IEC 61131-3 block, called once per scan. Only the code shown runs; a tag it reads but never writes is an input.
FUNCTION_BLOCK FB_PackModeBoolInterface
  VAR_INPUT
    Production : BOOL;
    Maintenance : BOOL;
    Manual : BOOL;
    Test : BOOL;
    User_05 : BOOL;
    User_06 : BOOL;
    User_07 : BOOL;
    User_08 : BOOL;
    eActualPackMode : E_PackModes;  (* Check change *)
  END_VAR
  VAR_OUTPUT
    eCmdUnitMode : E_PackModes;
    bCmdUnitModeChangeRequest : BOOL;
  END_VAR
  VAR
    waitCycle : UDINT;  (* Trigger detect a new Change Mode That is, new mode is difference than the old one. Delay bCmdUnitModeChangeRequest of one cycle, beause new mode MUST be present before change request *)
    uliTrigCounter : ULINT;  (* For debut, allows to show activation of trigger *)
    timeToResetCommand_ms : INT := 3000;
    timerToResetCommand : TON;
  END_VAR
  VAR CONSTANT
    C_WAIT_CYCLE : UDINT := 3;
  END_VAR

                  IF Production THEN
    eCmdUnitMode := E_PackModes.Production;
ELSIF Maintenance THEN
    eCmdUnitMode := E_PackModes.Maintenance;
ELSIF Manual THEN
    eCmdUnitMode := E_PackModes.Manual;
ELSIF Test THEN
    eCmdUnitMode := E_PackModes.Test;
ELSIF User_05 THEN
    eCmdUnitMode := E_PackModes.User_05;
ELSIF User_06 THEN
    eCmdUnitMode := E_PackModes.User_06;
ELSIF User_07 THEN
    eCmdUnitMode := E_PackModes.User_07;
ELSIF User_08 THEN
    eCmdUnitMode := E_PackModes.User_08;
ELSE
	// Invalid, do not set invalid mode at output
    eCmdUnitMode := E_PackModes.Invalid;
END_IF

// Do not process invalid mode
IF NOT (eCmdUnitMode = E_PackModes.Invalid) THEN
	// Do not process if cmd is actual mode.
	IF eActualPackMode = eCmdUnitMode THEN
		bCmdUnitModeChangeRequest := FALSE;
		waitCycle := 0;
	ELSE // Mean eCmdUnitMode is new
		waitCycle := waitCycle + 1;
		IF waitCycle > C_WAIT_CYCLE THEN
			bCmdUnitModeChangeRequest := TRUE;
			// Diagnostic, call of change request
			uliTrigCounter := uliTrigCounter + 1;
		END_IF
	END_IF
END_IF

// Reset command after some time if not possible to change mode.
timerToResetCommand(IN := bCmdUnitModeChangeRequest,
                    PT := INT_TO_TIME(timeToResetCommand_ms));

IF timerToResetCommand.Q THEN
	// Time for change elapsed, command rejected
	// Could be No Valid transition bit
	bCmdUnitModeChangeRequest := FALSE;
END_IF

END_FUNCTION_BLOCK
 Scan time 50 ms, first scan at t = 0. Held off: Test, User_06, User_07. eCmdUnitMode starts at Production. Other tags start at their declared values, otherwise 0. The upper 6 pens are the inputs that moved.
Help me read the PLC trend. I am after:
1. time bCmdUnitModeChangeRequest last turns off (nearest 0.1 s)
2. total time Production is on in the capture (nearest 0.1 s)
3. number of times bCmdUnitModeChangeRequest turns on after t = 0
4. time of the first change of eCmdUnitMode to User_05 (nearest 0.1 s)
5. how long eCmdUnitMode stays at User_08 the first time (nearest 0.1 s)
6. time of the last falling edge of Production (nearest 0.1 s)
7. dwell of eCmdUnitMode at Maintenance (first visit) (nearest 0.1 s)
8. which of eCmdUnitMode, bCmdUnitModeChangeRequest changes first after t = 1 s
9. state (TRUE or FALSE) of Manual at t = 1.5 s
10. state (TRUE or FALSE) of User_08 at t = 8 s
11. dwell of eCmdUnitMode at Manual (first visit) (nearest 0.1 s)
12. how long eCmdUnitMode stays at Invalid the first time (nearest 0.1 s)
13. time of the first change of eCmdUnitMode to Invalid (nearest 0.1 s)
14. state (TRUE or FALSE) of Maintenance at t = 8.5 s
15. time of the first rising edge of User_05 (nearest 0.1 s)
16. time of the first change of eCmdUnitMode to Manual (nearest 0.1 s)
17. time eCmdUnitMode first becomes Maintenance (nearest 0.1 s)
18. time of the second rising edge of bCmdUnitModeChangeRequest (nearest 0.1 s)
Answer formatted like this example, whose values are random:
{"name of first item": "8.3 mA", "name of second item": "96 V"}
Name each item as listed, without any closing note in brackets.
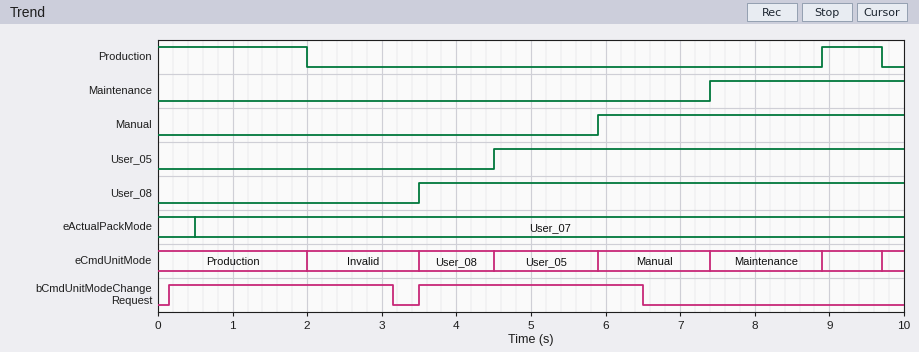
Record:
{"time bCmdUnitModeChangeRequest last turns off": "6.5 s", "total time Production is on in the capture": "2.8 s", "number of times bCmdUnitModeChangeRequest turns on after t = 0": "2", "time of the first change of eCmdUnitMode to User_05": "4.5 s", "how long eCmdUnitMode stays at User_08 the first time": "1.0 s", "time of the last falling edge of Production": "9.7 s", "dwell of eCmdUnitMode at Maintenance (first visit)": "1.5 s", "which of eCmdUnitMode, bCmdUnitModeChangeRequest changes first after t = 1 s": "eCmdUnitMode", "state (TRUE or FALSE) of Manual at t = 1.5 s": "FALSE", "state (TRUE or FALSE) of User_08 at t = 8 s": "TRUE", "dwell of eCmdUnitMode at Manual (first visit)": "1.5 s", "how long eCmdUnitMode stays at Invalid the first time": "1.5 s", "time of the first change of eCmdUnitMode to Invalid": "2.0 s", "state (TRUE or FALSE) of Maintenance at t = 8.5 s": "TRUE", "time of the first rising edge of User_05": "4.5 s", "time of the first change of eCmdUnitMode to Manual": "5.9 s", "time eCmdUnitMode first becomes Maintenance": "7.4 s", "time of the second rising edge of bCmdUnitModeChangeRequest": "3.5 s"}
